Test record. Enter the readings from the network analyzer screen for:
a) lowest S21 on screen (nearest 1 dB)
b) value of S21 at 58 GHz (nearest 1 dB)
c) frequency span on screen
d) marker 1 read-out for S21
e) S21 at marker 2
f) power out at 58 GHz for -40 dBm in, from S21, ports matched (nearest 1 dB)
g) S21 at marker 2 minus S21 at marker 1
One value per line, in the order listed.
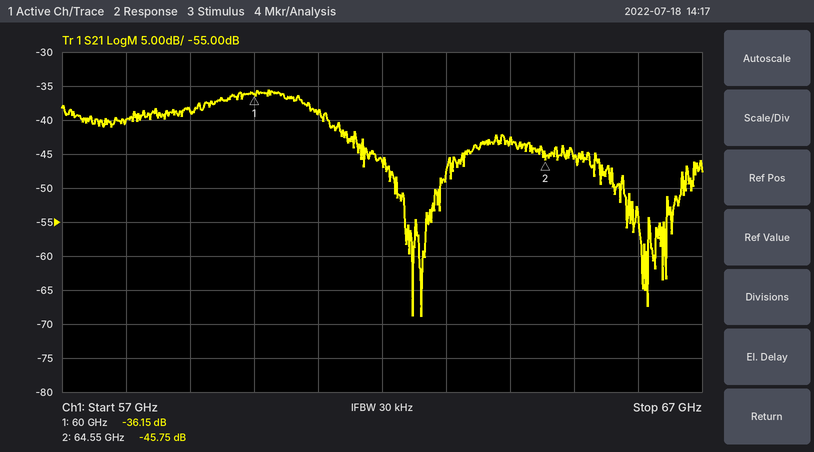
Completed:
-69 dB
-40 dB
10 GHz
-36.15 dB
-45.75 dB
-80 dBm
-9.60 dB
